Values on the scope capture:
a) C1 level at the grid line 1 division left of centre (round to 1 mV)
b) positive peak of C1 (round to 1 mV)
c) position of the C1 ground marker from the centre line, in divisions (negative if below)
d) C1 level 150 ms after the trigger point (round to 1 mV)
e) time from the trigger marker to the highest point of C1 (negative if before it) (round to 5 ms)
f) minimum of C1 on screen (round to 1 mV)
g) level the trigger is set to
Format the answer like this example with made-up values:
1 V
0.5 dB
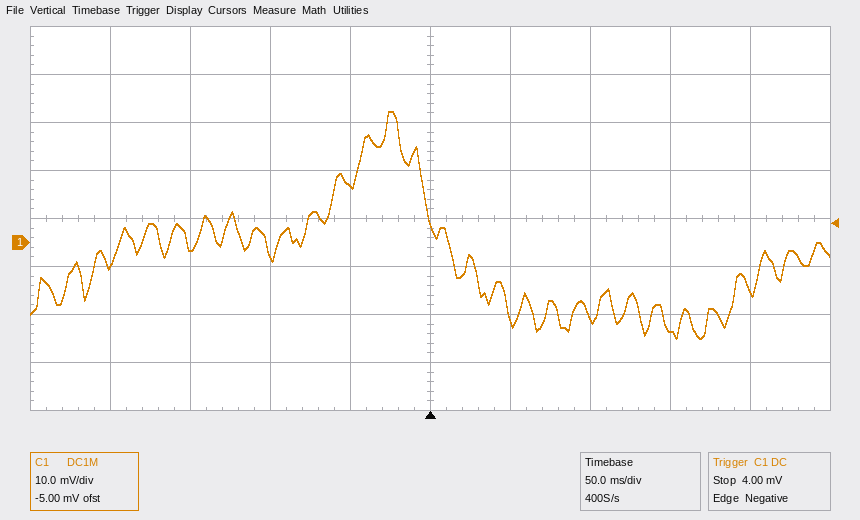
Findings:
12 mV
27 mV
-0.5 div
-18 mV
-25 ms
-20 mV
4.00 mV
